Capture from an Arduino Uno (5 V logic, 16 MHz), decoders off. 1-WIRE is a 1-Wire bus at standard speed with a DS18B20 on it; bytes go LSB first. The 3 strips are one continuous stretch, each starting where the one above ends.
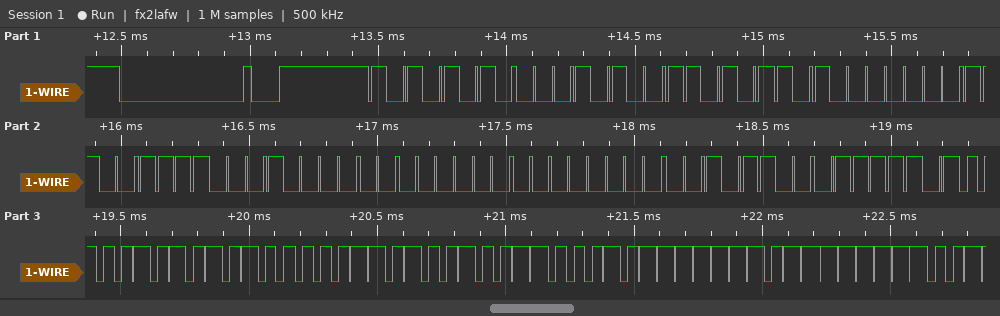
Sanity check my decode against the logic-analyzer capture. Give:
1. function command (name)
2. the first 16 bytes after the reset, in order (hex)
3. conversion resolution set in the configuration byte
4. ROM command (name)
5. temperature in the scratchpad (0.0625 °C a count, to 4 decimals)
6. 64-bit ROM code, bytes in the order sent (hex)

Read Scratchpad
55 28 6B 01 F3 08 00 00 34 BE 50 05 4B 46 7F FF
12 bits
Match ROM
85.0000 °C
28 6B 01 F3 08 00 00 34
